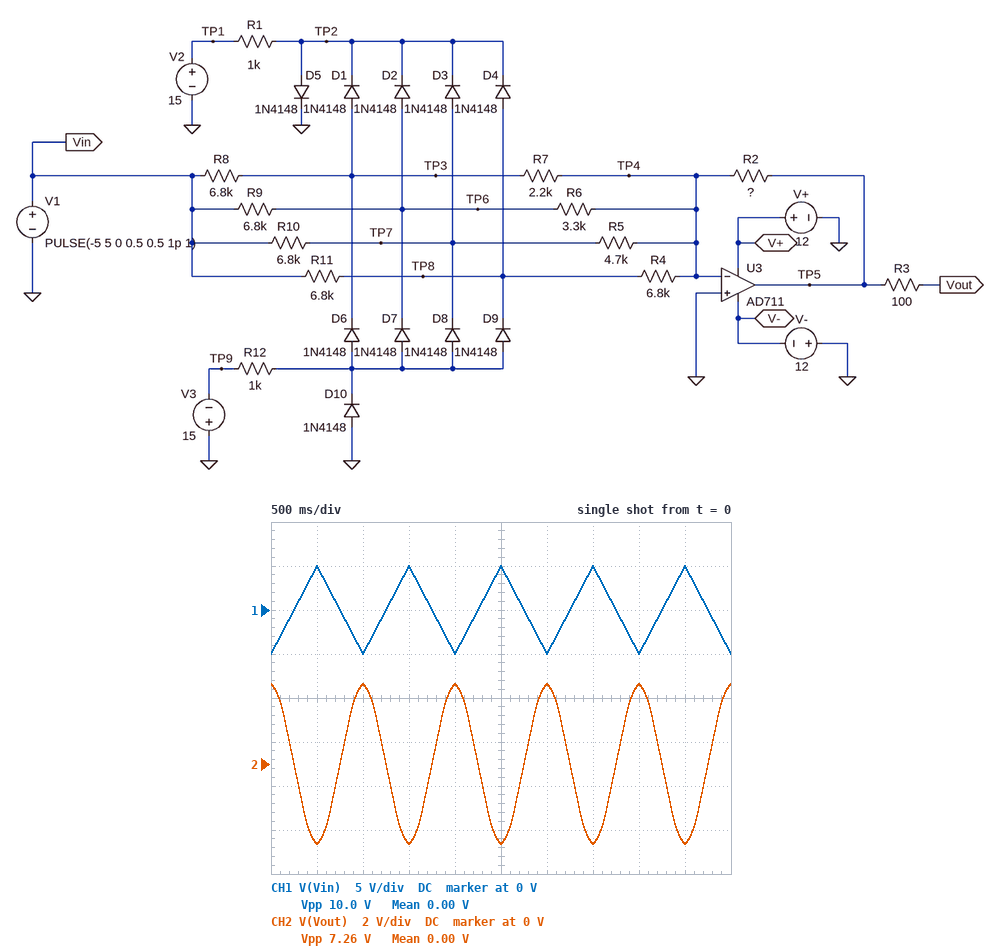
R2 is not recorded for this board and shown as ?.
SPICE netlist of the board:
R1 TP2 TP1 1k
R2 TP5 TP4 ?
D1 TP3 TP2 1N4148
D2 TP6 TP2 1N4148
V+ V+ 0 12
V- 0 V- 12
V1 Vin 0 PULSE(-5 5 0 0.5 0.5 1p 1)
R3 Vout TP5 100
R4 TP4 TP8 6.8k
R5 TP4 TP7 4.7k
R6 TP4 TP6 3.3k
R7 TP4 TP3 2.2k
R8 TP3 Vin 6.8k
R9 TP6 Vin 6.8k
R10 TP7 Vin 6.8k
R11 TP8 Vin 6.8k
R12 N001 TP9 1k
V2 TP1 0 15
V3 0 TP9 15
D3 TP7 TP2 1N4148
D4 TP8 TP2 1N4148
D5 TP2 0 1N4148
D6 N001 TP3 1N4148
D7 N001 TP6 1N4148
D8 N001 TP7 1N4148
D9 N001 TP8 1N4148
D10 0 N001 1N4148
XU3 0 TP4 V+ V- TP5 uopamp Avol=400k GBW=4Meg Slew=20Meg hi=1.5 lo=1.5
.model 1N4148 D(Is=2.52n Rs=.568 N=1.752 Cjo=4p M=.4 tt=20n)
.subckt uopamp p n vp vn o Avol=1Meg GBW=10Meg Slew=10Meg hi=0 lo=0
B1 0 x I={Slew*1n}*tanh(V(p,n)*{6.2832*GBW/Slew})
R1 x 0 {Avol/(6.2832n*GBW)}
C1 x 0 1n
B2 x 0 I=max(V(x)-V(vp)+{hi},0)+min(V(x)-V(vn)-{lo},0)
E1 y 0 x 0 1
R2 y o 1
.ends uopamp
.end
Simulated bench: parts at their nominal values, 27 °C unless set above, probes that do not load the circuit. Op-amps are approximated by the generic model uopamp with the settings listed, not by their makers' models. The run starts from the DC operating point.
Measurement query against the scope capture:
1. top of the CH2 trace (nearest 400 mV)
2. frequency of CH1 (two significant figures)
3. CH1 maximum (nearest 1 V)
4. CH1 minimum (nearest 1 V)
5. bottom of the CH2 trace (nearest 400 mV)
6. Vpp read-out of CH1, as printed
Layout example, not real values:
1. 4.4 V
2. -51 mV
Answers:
1. 3.6 V
2. 1.0 Hz
3. 5 V
4. -5 V
5. -3.6 V
6. 10.0 V
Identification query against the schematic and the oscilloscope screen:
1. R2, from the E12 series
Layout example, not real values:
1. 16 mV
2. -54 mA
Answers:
1. 2.7 kΩ
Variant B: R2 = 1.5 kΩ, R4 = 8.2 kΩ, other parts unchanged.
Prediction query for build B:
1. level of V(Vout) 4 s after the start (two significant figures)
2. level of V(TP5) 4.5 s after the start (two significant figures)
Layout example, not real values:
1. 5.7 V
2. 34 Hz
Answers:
1. 2.0 V
2. -2.0 V
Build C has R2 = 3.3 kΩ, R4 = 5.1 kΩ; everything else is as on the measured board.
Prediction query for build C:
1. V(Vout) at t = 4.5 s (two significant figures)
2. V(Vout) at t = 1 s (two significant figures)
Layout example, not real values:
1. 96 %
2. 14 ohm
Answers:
1. -4.6 V
2. 4.6 V
